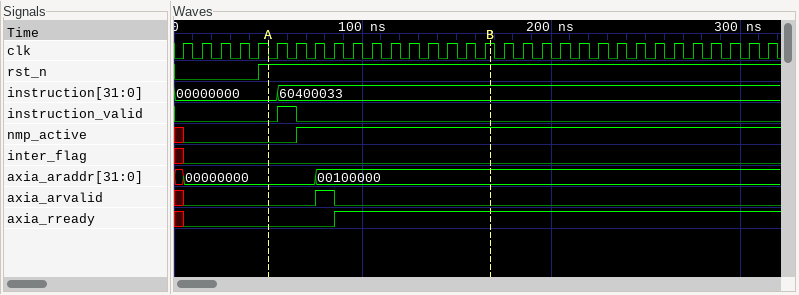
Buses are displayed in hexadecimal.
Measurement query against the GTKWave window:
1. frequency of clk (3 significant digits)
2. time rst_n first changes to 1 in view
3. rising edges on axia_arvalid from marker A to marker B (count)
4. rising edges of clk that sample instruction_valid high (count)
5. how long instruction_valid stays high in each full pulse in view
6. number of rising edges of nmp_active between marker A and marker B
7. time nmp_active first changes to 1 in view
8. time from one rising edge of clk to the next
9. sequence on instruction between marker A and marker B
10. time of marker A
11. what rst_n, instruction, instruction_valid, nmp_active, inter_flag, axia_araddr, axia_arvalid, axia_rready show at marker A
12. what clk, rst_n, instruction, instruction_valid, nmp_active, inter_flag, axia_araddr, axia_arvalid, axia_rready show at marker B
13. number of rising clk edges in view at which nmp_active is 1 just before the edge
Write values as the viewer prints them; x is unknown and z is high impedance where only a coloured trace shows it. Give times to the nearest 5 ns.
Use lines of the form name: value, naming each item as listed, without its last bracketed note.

frequency of clk: 100 MHz
time rst_n first changes to 1 in view: 45 ns
rising edges on axia_arvalid from marker A to marker B: 1
rising edges of clk that sample instruction_valid high: 1
how long instruction_valid stays high in each full pulse in view: 10 ns
number of rising edges of nmp_active between marker A and marker B: 1
time nmp_active first changes to 1 in view: 65 ns
time from one rising edge of clk to the next: 10 ns
sequence on instruction between marker A and marker B: 00000000, 60400033
time of marker A: 50 ns
what rst_n, instruction, instruction_valid, nmp_active, inter_flag, axia_araddr, axia_arvalid, axia_rready show at marker A: rst_n=1, instruction=00000000, instruction_valid=0, nmp_active=0, inter_flag=0, axia_araddr=00000000, axia_arvalid=0, axia_rready=0
what clk, rst_n, instruction, instruction_valid, nmp_active, inter_flag, axia_araddr, axia_arvalid, axia_rready show at marker B: clk=1, rst_n=1, instruction=60400033, instruction_valid=0, nmp_active=1, inter_flag=0, axia_araddr=00100000, axia_arvalid=0, axia_rready=1
number of rising clk edges in view at which nmp_active is 1 just before the edge: 25
